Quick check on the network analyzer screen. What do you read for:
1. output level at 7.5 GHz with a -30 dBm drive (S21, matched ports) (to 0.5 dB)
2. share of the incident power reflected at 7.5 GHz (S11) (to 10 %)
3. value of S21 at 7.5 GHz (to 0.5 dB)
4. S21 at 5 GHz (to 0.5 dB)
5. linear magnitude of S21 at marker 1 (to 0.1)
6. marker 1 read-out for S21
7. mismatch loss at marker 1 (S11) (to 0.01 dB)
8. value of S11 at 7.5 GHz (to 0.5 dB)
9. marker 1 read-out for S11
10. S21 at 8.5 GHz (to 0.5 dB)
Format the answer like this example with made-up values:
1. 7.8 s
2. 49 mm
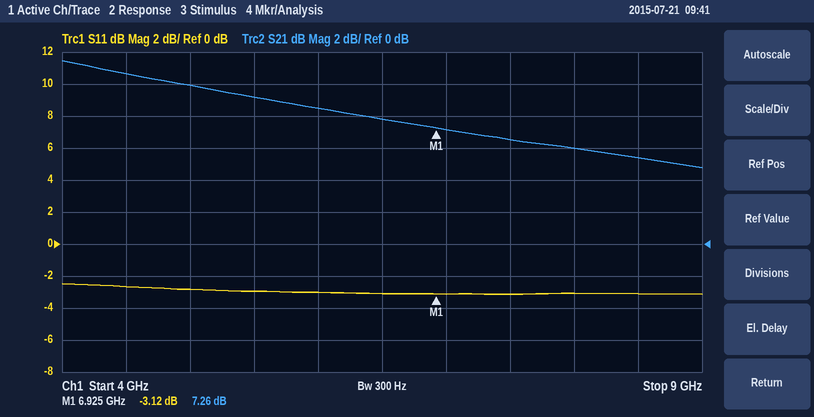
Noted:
1. -23.5 dBm
2. 50 %
3. 6.5 dB
4. 10.0 dB
5. 2.3
6. 7.26 dB
7. 2.90 dB
8. -3.0 dB
9. -3.12 dB
10. 5.5 dB
